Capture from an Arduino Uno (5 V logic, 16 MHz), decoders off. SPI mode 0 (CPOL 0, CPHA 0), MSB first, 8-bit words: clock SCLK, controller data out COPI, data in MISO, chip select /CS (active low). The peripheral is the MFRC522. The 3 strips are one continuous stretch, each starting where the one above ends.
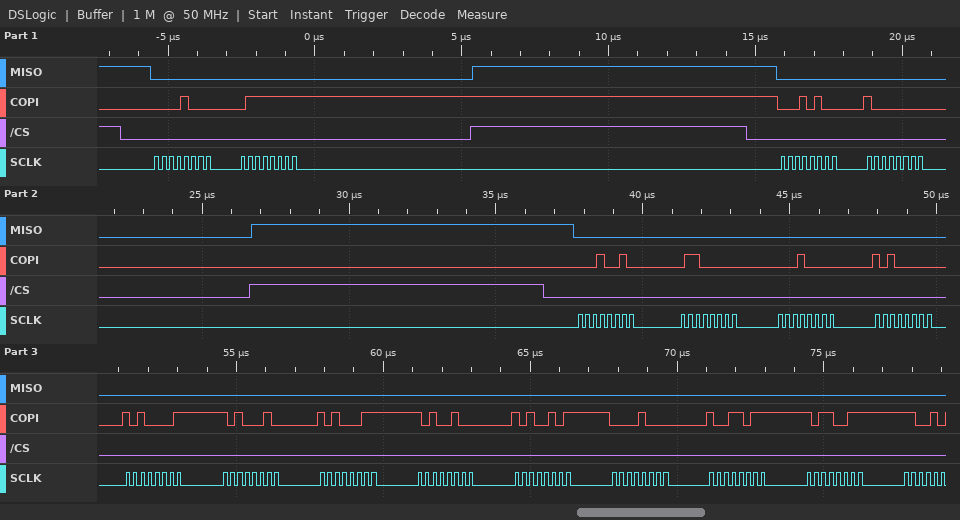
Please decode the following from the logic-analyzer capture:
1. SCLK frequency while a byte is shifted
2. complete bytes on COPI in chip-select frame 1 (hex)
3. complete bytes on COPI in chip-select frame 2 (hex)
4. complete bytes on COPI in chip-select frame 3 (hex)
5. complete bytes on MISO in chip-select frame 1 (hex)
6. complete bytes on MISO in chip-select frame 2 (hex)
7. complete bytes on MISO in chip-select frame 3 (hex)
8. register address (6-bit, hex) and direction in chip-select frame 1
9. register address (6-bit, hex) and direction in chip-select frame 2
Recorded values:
4 MHz
08 7F
14 80
12 60 10 A0 A1 A2 A3 A4 A5 08 9B B3
00 00
00 00
00 00 00 00 00 00 00 00 00 00 00 00
0x04 write
0x0A write
